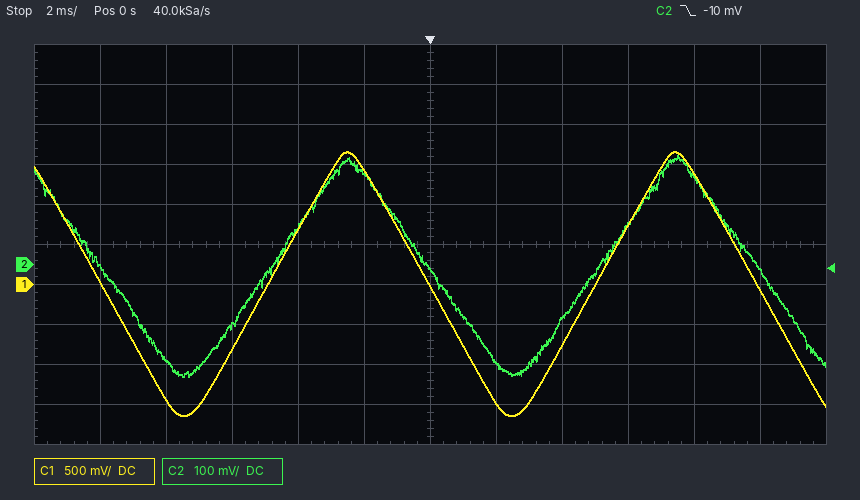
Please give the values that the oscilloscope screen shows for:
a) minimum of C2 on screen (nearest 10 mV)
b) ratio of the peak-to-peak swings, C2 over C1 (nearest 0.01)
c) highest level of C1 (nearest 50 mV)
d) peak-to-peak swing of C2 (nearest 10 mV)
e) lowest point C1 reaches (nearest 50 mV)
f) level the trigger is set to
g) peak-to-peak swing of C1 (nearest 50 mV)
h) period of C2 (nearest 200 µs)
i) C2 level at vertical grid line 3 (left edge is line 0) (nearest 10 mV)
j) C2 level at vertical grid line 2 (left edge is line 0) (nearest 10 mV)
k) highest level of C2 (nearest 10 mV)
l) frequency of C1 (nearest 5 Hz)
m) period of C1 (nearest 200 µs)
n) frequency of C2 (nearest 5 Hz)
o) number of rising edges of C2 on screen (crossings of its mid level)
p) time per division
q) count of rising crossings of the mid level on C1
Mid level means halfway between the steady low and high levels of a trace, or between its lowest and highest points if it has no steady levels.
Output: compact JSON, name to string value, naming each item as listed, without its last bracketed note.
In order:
{"minimum of C2 on screen": "-280 mV", "ratio of the peak-to-peak swings, C2 over C1": "0.17", "highest level of C1": "1.65 V", "peak-to-peak swing of C2": "550 mV", "lowest point C1 reaches": "-1.65 V", "level the trigger is set to": "-10 mV", "peak-to-peak swing of C1": "3.30 V", "period of C2": "10.0 ms", "C2 level at vertical grid line 3 (left edge is line 0)": "-150 mV", "C2 level at vertical grid line 2 (left edge is line 0)": "-240 mV", "highest level of C2": "270 mV", "frequency of C1": "100 Hz", "period of C1": "10.0 ms", "frequency of C2": "100 Hz", "number of rising edges of C2 on screen": "2", "time per division": "2 ms", "count of rising crossings of the mid level on C1": "2"}
